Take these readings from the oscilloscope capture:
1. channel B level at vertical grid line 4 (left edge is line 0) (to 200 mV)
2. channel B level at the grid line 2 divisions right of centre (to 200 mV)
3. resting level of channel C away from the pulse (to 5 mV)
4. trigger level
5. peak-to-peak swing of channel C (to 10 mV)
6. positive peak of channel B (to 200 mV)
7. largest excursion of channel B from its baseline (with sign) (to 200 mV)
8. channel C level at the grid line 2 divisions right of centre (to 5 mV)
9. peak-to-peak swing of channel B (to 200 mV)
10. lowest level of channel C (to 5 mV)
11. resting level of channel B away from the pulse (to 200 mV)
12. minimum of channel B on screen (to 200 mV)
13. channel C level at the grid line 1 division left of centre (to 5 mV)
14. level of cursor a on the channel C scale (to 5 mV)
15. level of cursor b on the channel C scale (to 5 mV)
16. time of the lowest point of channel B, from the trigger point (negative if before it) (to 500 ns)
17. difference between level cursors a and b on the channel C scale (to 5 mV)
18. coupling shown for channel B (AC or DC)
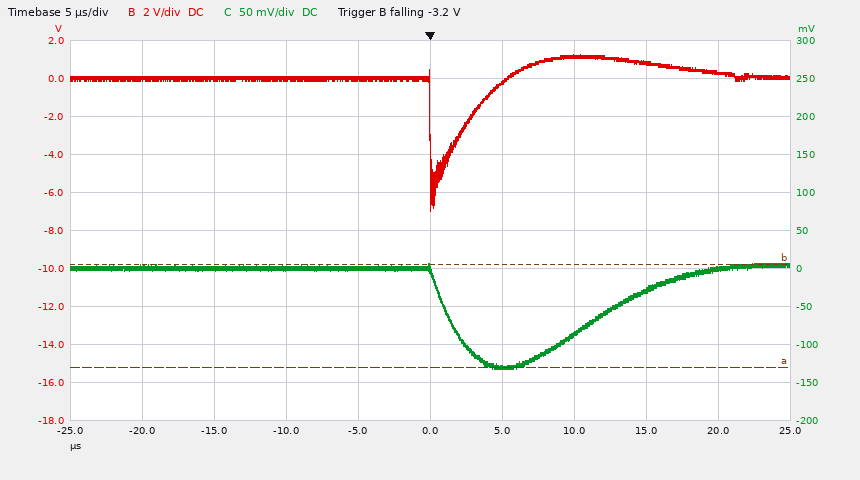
0.0 V
1.2 V
0 mV
-3.2 V
140 mV
1.2 V
-7.0 V
-85 mV
8.2 V
-130 mV
0.0 V
-7.0 V
0 mV
-130 mV
5 mV
0.0 µs
135 mV
DC
